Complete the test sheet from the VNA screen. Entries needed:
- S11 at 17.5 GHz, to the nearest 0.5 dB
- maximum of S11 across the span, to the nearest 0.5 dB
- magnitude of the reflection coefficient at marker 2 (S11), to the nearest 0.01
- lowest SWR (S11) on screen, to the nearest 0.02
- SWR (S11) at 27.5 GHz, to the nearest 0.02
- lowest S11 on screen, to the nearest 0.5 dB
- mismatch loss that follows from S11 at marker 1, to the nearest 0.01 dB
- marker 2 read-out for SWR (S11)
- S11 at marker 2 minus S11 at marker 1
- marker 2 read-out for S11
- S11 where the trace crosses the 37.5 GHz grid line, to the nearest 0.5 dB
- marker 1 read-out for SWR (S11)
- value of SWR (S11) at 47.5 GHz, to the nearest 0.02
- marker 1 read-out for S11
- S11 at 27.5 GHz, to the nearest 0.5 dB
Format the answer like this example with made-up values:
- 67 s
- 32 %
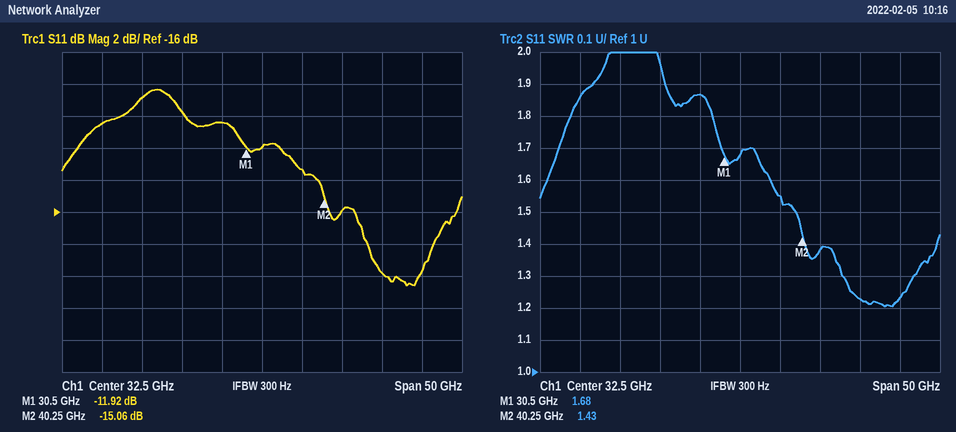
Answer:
- -9.0 dB
- -8.5 dB
- 0.18
- 1.20
- 1.86
- -20.5 dB
- 0.29 dB
- 1.43
- -3.14 dB
- -15.06 dB
- -13.5 dB
- 1.68
- 1.22
- -11.92 dB
- -10.5 dB
